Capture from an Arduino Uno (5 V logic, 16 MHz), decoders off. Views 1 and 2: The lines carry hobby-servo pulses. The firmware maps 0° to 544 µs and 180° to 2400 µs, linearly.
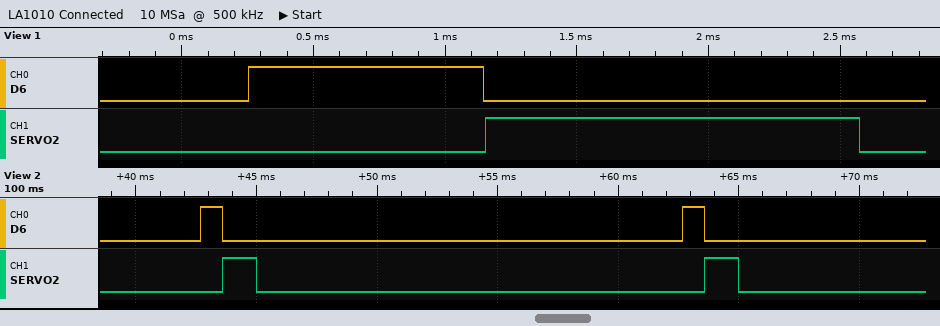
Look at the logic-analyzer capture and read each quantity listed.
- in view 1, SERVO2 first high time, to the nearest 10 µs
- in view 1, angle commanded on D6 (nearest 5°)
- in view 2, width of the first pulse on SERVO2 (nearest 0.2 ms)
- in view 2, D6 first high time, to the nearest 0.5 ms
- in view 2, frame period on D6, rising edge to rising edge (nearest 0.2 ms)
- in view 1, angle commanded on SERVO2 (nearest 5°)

1420 µs
35°
1.4 ms
1.0 ms
20.0 ms
85°
